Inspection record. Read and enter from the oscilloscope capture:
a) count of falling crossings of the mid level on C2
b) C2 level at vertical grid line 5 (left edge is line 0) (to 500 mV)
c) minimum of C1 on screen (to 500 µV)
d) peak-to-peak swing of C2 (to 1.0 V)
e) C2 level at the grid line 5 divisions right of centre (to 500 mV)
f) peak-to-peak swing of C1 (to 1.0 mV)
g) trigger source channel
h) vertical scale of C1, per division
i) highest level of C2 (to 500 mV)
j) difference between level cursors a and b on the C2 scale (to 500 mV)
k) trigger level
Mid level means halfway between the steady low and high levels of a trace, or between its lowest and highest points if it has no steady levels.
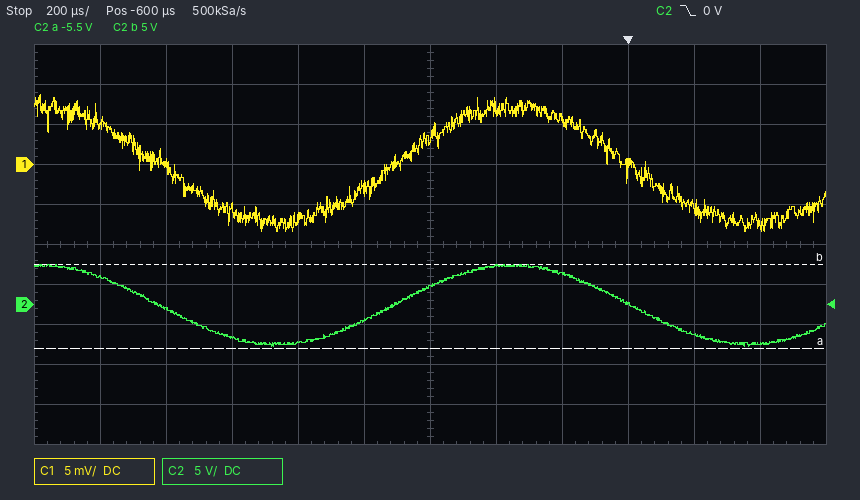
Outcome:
2
-2.0 V
-8.5 mV
10.0 V
-5.0 V
17.0 mV
C2
5 mV
5.0 V
10.5 V
0 V
